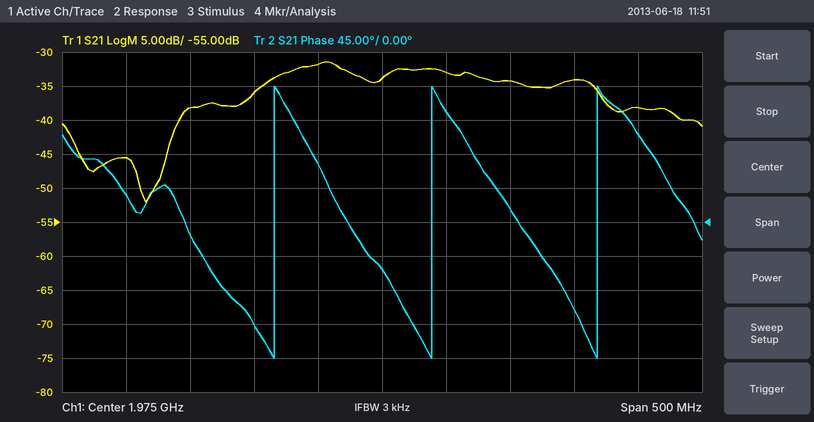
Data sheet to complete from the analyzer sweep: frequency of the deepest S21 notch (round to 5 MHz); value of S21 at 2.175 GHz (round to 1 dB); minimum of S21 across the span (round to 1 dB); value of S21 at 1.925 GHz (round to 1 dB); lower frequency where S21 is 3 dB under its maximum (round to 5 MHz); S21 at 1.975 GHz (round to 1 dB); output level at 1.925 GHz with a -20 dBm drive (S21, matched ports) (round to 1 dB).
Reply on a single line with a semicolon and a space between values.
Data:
1.790 GHz; -38 dB; -52 dB; -32 dB; 1.885 GHz; -34 dB; -52 dBm
